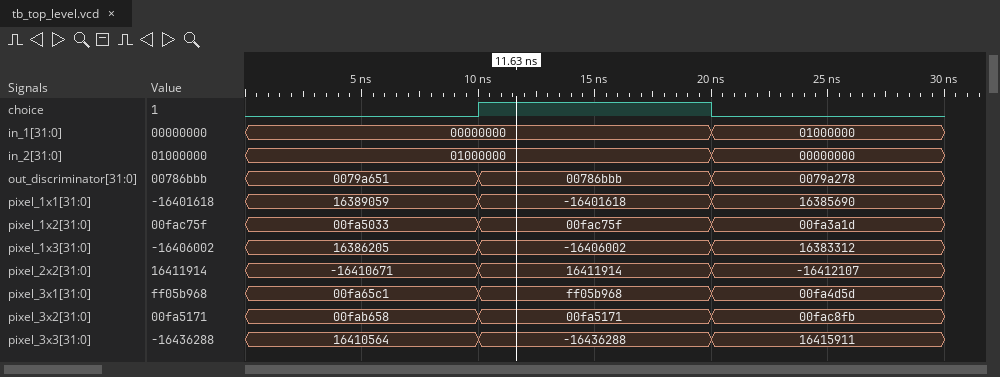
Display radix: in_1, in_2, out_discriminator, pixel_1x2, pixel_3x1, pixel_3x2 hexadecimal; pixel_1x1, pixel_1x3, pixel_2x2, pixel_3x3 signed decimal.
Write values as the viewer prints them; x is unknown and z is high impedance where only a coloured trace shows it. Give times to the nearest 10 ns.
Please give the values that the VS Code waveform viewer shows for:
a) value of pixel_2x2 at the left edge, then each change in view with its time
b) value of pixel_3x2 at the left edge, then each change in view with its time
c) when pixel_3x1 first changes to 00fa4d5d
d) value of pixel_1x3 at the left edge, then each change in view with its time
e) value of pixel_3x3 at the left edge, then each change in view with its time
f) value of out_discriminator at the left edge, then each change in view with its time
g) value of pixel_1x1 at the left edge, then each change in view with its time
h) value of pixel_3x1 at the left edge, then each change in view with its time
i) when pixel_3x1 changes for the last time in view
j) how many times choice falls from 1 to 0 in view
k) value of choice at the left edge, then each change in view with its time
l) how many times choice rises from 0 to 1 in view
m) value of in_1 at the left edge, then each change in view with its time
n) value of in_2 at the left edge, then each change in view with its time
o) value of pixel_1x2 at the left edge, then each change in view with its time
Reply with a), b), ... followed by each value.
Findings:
a) -16410671, 16411914 at 10 ns, -16412107 at 20 ns
b) 00fab658, 00fa5171 at 10 ns, 00fac8fb at 20 ns
c) 20 ns
d) 16386205, -16406002 at 10 ns, 16383312 at 20 ns
e) 16410564, -16436288 at 10 ns, 16415911 at 20 ns
f) 0079a651, 00786bbb at 10 ns, 0079a278 at 20 ns
g) 16389059, -16401618 at 10 ns, 16385690 at 20 ns
h) 00fa65c1, ff05b968 at 10 ns, 00fa4d5d at 20 ns
i) 20 ns
j) 1
k) 0, 1 at 10 ns, 0 at 20 ns
l) 1
m) 00000000, 01000000 at 20 ns
n) 01000000, 00000000 at 20 ns
o) 00fa5033, 00fac75f at 10 ns, 00fa3a1d at 20 ns
